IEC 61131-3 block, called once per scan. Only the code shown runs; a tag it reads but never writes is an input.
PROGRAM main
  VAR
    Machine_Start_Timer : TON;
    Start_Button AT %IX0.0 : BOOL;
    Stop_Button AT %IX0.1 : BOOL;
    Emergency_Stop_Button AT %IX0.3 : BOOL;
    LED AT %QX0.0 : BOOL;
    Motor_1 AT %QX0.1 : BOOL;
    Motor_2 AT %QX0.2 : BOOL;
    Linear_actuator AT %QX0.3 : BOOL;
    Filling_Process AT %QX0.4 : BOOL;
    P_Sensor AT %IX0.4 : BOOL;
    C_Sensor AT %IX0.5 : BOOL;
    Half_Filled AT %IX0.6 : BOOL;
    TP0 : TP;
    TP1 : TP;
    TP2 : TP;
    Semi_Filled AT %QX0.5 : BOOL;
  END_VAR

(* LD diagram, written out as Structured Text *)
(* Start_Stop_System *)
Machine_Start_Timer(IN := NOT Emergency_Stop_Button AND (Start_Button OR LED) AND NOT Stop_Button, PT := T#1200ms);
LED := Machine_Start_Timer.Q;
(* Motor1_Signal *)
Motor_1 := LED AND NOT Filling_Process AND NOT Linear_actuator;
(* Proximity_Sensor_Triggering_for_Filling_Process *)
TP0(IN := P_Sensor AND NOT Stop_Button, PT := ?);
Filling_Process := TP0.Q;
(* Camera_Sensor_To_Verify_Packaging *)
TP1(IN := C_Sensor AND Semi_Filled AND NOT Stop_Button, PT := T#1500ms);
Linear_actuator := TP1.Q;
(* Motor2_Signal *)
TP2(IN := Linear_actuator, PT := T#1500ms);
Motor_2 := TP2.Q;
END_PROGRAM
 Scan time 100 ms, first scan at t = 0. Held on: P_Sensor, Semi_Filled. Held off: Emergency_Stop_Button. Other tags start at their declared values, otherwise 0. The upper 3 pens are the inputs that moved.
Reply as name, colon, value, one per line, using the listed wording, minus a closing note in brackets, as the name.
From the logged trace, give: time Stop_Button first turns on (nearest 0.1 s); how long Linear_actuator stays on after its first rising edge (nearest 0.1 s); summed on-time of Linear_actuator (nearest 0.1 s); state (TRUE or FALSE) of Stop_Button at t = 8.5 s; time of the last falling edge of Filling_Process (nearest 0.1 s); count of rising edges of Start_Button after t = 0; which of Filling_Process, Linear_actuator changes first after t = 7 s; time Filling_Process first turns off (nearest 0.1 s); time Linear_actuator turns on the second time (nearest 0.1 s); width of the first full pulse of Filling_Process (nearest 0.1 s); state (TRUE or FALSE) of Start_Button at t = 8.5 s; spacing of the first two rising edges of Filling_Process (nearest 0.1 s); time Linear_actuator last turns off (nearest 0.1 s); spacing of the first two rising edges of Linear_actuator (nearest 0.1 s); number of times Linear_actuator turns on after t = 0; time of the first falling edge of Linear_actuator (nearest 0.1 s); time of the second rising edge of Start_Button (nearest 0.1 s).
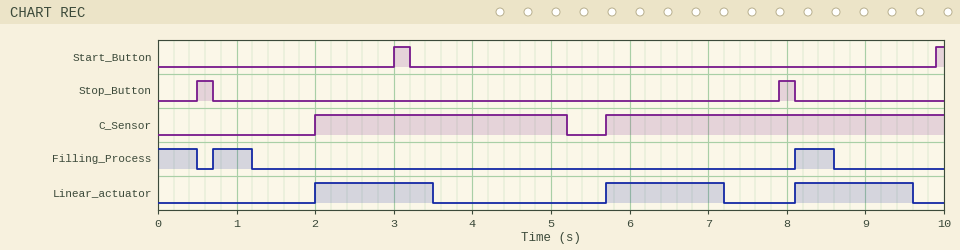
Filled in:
time Stop_Button first turns on: 0.5 s
how long Linear_actuator stays on after its first rising edge: 1.5 s
summed on-time of Linear_actuator: 4.5 s
state (TRUE or FALSE) of Stop_Button at t = 8.5 s: FALSE
time of the last falling edge of Filling_Process: 8.6 s
count of rising edges of Start_Button after t = 0: 2
which of Filling_Process, Linear_actuator changes first after t = 7 s: Linear_actuator
time Filling_Process first turns off: 0.5 s
time Linear_actuator turns on the second time: 5.7 s
width of the first full pulse of Filling_Process: 0.5 s
state (TRUE or FALSE) of Start_Button at t = 8.5 s: FALSE
spacing of the first two rising edges of Filling_Process: 7.4 s
time Linear_actuator last turns off: 9.6 s
spacing of the first two rising edges of Linear_actuator: 3.7 s
number of times Linear_actuator turns on after t = 0: 3
time of the first falling edge of Linear_actuator: 3.5 s
time of the second rising edge of Start_Button: 9.9 s
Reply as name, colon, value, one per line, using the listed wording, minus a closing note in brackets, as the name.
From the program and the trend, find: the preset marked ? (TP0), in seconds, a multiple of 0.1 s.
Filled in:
the preset marked ? (TP0), in seconds, a multiple of 0.1 s: 0.5 s
